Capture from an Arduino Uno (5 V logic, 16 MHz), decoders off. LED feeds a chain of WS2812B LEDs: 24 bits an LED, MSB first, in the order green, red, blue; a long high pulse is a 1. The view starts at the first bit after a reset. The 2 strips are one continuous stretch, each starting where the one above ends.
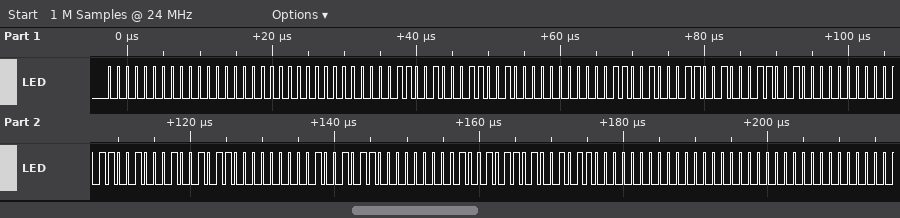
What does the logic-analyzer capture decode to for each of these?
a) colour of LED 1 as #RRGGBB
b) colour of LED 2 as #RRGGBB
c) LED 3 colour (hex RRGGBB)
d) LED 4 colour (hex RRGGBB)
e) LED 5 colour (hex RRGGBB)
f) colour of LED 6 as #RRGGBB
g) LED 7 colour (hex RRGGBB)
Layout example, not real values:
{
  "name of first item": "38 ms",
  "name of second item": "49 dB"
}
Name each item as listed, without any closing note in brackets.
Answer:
{
  "colour of LED 1 as #RRGGBB": "#000000",
  "colour of LED 2 as #RRGGBB": "#C800C8",
  "LED 3 colour": "#C800C8",
  "LED 4 colour": "#00C8C8",
  "LED 5 colour": "#009696",
  "colour of LED 6 as #RRGGBB": "#960096",
  "LED 7 colour": "#000000"
}
